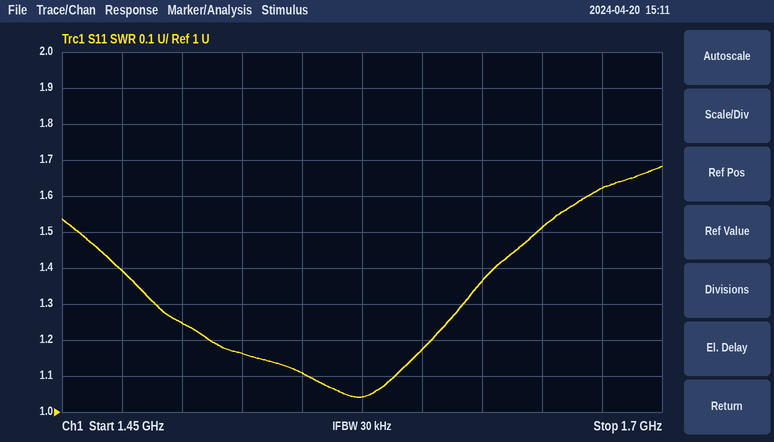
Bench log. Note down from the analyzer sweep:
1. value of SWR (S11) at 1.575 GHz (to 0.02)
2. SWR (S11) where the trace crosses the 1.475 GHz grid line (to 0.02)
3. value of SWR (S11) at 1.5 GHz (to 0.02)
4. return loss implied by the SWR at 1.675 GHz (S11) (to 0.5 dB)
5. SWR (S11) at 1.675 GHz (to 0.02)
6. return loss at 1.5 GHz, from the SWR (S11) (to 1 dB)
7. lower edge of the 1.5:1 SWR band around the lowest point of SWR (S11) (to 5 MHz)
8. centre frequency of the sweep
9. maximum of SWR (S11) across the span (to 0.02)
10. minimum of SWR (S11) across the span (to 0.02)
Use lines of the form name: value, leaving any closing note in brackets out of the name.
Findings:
value of SWR (S11) at 1.575 GHz: 1.04
SWR (S11) where the trace crosses the 1.475 GHz grid line: 1.40
value of SWR (S11) at 1.5 GHz: 1.24
return loss implied by the SWR at 1.675 GHz (S11): 12.5 dB
SWR (S11) at 1.675 GHz: 1.62
return loss at 1.5 GHz, from the SWR (S11): 19 dB
lower edge of the 1.5:1 SWR band around the lowest point of SWR (S11): 1.455 GHz
centre frequency of the sweep: 1.575 GHz
maximum of SWR (S11) across the span: 1.68
minimum of SWR (S11) across the span: 1.04
